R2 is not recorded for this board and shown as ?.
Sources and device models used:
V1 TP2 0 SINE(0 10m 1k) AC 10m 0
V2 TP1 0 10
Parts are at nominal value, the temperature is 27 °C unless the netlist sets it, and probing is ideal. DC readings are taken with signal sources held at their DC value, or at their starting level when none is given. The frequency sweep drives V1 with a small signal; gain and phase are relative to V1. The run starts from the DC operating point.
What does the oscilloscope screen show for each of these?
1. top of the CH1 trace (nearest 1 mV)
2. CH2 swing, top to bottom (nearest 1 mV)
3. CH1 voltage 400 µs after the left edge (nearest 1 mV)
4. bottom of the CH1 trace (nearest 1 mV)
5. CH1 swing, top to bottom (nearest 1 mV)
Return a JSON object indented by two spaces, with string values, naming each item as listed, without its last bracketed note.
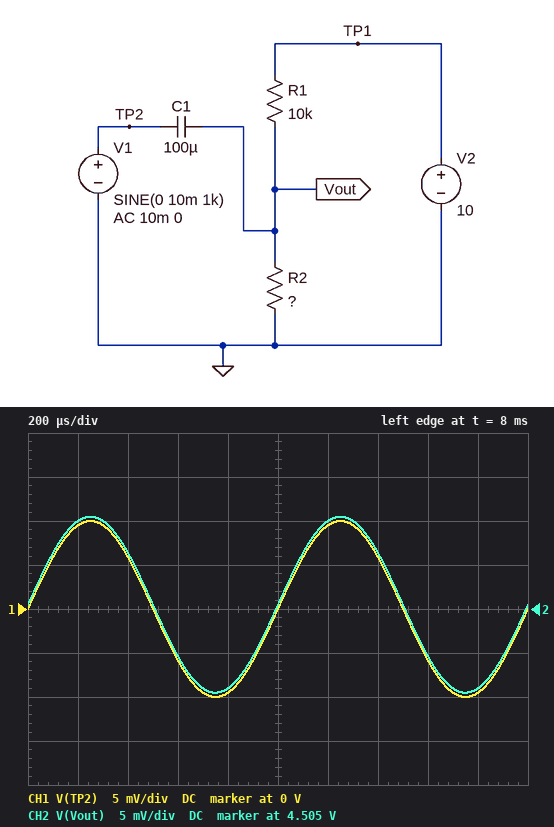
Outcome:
{
  "top of the CH1 trace": "10 mV",
  "CH2 swing, top to bottom": "20 mV",
  "CH1 voltage 400 µs after the left edge": "6 mV",
  "bottom of the CH1 trace": "-10 mV",
  "CH1 swing, top to bottom": "20 mV"
}
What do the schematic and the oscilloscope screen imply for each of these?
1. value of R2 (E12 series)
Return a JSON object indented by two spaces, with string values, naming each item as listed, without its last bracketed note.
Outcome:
{
  "value of R2": "8.2 kΩ"
}
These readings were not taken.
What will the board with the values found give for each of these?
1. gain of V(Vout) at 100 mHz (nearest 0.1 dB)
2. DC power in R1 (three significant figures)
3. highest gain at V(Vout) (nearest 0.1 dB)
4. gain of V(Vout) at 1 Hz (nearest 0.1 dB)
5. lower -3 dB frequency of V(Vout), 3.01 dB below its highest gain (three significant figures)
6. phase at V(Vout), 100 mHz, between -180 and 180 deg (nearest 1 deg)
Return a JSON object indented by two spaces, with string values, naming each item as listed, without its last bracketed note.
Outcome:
{
  "gain of V(Vout) at 100 mHz": "-11.3 dB",
  "DC power in R1": "3.02 mW",
  "highest gain at V(Vout)": "0 dB",
  "gain of V(Vout) at 1 Hz": "-0.5 dB",
  "lower -3 dB frequency of V(Vout), 3.01 dB below its highest gain": "353 mHz",
  "phase at V(Vout), 100 mHz, between -180 and 180 deg": "74 deg"
}
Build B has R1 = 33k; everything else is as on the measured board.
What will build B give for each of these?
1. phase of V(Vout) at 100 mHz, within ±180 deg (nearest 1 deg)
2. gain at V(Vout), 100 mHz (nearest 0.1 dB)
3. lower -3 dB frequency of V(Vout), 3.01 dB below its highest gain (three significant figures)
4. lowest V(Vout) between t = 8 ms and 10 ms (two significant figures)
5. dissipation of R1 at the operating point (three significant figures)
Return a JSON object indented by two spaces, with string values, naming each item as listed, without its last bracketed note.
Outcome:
{
  "phase of V(Vout) at 100 mHz, within ±180 deg": "68 deg",
  "gain at V(Vout), 100 mHz": "-8.4 dB",
  "lower -3 dB frequency of V(Vout), 3.01 dB below its highest gain": "242 mHz",
  "lowest V(Vout) between t = 8 ms and 10 ms": "2.0 V",
  "dissipation of R1 at the operating point": "1.94 mW"
}
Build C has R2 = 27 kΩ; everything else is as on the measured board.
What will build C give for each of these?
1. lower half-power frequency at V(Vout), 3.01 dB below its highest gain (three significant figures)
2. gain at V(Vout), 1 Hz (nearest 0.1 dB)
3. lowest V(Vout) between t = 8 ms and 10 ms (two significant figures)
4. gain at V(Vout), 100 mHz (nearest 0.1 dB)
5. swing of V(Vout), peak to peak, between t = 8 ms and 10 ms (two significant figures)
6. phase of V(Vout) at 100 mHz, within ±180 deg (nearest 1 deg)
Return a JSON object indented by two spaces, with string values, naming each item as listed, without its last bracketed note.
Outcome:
{
  "lower half-power frequency at V(Vout), 3.01 dB below its highest gain": "218 mHz",
  "gain at V(Vout), 1 Hz": "-0.2 dB",
  "lowest V(Vout) between t = 8 ms and 10 ms": "7.3 V",
  "gain at V(Vout), 100 mHz": "-7.6 dB",
  "swing of V(Vout), peak to peak, between t = 8 ms and 10 ms": "20 mV",
  "phase of V(Vout) at 100 mHz, within ±180 deg": "65 deg"
}
